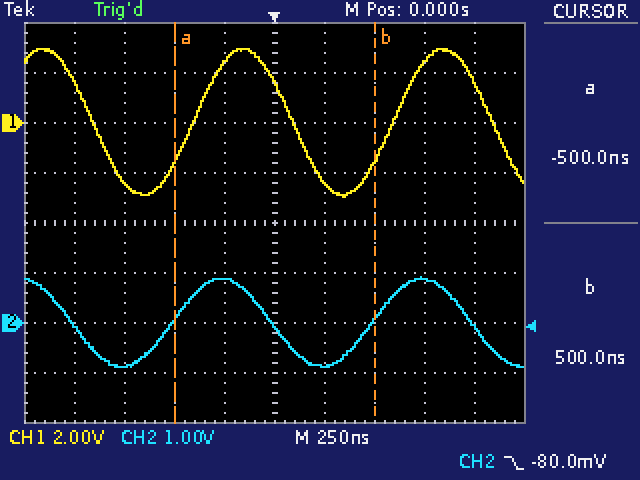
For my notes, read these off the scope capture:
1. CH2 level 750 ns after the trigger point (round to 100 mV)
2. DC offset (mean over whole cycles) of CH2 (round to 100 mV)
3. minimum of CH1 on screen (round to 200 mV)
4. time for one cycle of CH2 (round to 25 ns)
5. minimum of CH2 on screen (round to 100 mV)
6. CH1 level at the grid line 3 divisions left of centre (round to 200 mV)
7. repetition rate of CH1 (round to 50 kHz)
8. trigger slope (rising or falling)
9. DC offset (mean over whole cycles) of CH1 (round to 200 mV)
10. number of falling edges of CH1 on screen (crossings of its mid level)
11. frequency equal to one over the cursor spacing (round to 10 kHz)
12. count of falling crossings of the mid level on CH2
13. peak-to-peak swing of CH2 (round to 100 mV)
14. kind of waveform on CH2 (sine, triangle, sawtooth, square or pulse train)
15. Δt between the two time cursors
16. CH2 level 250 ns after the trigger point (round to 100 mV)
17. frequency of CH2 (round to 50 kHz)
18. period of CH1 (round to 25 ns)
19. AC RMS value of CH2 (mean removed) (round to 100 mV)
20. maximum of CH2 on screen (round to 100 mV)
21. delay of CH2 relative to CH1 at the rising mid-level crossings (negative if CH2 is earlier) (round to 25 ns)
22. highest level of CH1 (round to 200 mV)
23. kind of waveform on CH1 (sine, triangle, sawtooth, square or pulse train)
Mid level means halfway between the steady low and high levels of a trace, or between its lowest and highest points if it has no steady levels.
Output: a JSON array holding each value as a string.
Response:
["900 mV", "0.0 V", "-3.0 V", "1.000 µs", "-900 mV", "-2.4 V", "1.00 MHz", "falling", "0.0 V", "3", "1.00 MHz", "3", "1.8 V", "sine", "1.000 µs", "-900 mV", "1.00 MHz", "1.000 µs", "600 mV", "900 mV", "-100 ns", "3.0 V", "sine"]
